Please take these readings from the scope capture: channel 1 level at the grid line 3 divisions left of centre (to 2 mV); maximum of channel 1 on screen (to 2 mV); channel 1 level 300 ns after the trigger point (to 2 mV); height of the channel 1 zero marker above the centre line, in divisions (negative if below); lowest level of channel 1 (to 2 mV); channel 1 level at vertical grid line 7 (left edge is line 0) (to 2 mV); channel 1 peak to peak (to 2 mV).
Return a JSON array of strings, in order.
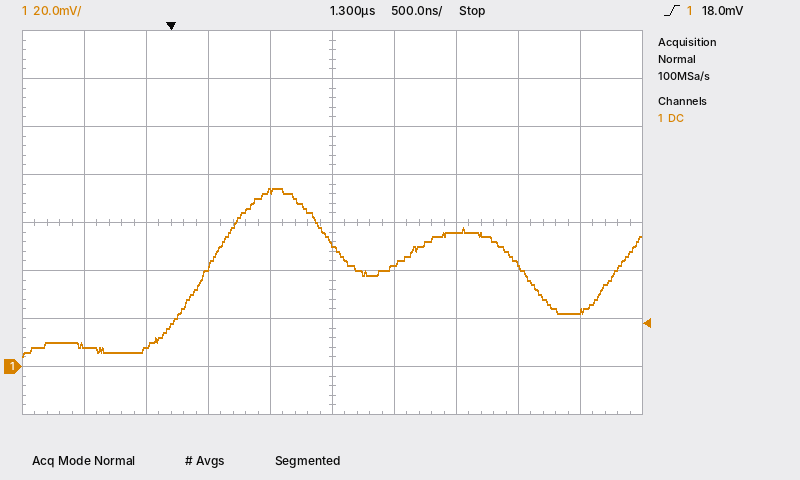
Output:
["8 mV", "74 mV", "42 mV", "-3.0 div", "4 mV", "56 mV", "70 mV"]
